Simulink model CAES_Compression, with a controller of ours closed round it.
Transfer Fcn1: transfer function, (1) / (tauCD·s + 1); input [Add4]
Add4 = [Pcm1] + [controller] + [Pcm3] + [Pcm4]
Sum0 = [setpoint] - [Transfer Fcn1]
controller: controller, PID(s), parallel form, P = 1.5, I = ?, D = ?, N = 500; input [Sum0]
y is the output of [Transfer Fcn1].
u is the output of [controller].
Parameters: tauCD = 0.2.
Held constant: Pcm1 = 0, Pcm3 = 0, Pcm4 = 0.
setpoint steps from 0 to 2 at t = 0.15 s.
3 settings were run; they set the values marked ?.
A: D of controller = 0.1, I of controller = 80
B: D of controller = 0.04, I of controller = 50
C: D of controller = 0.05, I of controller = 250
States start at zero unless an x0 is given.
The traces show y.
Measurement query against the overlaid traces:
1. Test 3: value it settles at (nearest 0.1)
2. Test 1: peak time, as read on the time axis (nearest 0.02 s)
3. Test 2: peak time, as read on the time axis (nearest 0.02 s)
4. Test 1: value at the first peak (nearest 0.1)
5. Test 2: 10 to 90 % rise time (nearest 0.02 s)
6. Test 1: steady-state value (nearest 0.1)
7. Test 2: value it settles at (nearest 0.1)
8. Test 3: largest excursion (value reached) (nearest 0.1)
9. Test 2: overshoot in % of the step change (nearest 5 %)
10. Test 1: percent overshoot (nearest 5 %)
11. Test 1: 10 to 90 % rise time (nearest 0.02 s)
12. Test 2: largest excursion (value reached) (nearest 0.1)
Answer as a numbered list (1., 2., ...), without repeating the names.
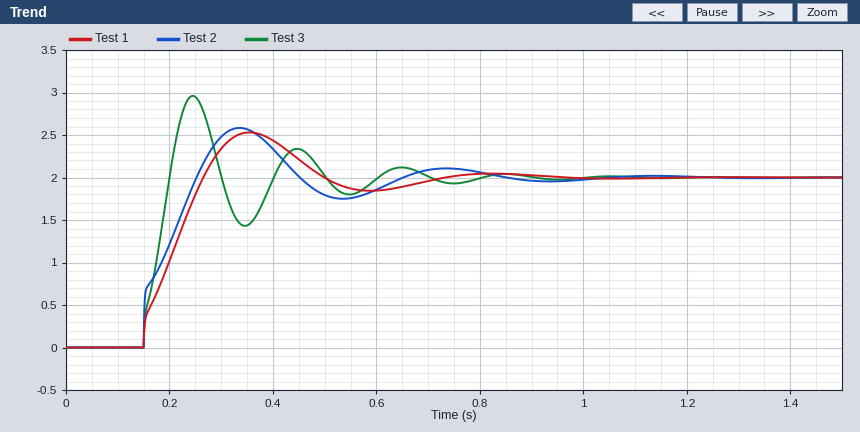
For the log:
1. 2.0
2. 0.36 s
3. 0.34 s
4. 2.5
5. 0.08 s
6. 2.0
7. 2.0
8. 3.0
9. 30 %
10. 25 %
11. 0.10 s
12. 2.6
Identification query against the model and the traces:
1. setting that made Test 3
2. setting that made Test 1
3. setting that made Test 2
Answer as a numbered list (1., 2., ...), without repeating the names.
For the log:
1. C
2. B
3. A
